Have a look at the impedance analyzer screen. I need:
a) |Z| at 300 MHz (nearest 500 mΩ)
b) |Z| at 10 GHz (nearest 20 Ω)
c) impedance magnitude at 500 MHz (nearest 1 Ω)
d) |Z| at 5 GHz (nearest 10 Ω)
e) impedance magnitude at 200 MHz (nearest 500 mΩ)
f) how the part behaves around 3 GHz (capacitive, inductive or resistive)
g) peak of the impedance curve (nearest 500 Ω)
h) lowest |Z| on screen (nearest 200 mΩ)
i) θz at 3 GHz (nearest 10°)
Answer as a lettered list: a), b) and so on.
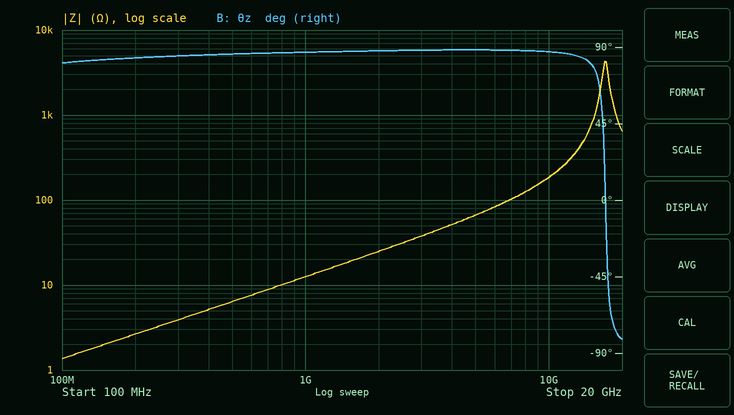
a) 4.0 Ω
b) 180 Ω
c) 6 Ω
d) 70 Ω
e) 2.5 Ω
f) inductive
g) 4.5 kΩ
h) 1.4 Ω
i) 90°
